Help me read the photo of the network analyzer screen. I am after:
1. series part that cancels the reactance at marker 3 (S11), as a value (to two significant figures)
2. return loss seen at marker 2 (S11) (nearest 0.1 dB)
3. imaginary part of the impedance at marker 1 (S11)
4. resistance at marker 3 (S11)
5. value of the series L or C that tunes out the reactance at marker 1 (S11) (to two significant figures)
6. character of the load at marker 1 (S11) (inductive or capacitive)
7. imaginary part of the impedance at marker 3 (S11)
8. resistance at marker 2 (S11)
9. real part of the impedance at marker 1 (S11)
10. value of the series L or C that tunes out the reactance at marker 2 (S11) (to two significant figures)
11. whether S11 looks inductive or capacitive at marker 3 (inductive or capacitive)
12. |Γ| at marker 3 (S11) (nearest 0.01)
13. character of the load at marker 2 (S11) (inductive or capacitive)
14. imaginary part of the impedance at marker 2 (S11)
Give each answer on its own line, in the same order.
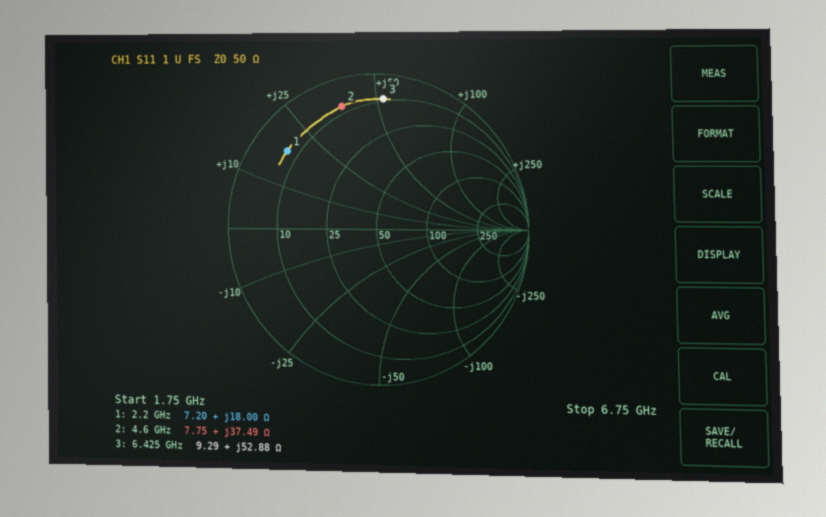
470 fF
1.7 dB
+18.00 Ω
9.29 Ω
4.0 pF
inductive
+52.88 Ω
7.75 Ω
7.20 Ω
920 fF
inductive
0.84
inductive
+37.49 Ω
